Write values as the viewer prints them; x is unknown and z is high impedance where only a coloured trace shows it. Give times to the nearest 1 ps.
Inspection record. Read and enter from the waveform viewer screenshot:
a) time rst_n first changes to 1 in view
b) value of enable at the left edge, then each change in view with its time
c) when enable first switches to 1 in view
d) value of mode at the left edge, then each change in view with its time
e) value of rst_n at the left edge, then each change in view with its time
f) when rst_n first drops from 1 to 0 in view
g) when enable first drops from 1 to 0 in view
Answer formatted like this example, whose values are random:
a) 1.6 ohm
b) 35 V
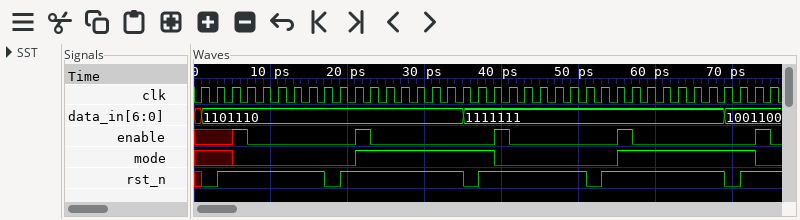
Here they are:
a) 3 ps
b) x, 1 at 5 ps, 0 at 7 ps, 1 at 21 ps, 0 at 23 ps, 1 at 39 ps, 0 at 41 ps, 1 at 55 ps, 0 at 57 ps, 1 at 73 ps, 0 at 75 ps
c) 5 ps
d) x, 0 at 5 ps, 1 at 21 ps, 0 at 39 ps, 1 at 55 ps, 0 at 73 ps
e) x, 0 at 1 ps, 1 at 3 ps, 0 at 17 ps, 1 at 19 ps, 0 at 35 ps, 1 at 37 ps, 0 at 51 ps, 1 at 53 ps, 0 at 69 ps, 1 at 71 ps
f) 17 ps
g) 7 ps
